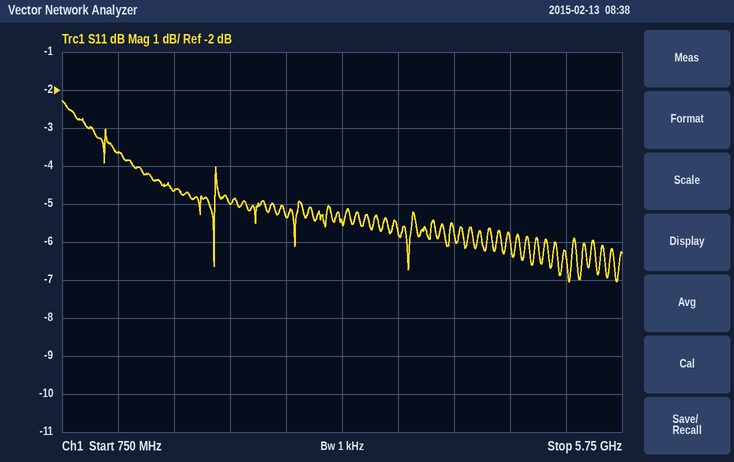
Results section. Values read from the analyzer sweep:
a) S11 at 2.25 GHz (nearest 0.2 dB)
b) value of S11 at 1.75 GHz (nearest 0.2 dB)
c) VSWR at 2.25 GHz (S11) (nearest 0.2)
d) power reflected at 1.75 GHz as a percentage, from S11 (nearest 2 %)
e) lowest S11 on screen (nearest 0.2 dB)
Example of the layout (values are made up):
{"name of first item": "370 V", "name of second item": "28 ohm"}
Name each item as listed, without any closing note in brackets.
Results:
{"S11 at 2.25 GHz": "-5.0 dB", "value of S11 at 1.75 GHz": "-4.6 dB", "VSWR at 2.25 GHz (S11)": "3.6", "power reflected at 1.75 GHz as a percentage, from S11": "34 %", "lowest S11 on screen": "-7.0 dB"}
